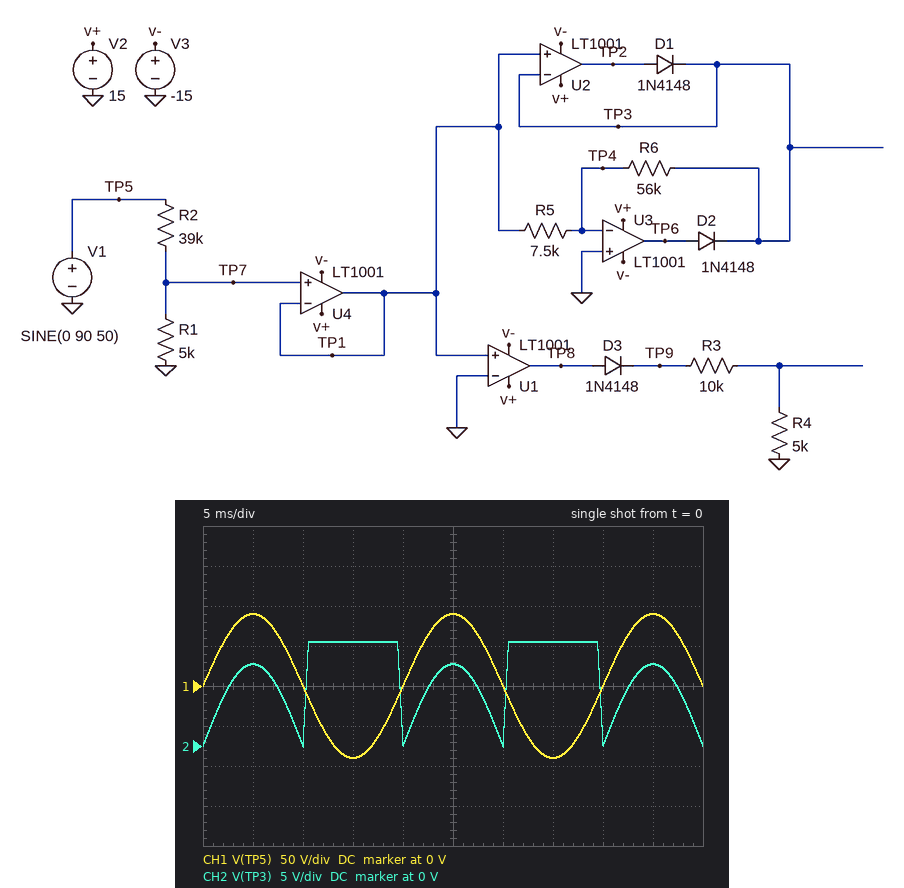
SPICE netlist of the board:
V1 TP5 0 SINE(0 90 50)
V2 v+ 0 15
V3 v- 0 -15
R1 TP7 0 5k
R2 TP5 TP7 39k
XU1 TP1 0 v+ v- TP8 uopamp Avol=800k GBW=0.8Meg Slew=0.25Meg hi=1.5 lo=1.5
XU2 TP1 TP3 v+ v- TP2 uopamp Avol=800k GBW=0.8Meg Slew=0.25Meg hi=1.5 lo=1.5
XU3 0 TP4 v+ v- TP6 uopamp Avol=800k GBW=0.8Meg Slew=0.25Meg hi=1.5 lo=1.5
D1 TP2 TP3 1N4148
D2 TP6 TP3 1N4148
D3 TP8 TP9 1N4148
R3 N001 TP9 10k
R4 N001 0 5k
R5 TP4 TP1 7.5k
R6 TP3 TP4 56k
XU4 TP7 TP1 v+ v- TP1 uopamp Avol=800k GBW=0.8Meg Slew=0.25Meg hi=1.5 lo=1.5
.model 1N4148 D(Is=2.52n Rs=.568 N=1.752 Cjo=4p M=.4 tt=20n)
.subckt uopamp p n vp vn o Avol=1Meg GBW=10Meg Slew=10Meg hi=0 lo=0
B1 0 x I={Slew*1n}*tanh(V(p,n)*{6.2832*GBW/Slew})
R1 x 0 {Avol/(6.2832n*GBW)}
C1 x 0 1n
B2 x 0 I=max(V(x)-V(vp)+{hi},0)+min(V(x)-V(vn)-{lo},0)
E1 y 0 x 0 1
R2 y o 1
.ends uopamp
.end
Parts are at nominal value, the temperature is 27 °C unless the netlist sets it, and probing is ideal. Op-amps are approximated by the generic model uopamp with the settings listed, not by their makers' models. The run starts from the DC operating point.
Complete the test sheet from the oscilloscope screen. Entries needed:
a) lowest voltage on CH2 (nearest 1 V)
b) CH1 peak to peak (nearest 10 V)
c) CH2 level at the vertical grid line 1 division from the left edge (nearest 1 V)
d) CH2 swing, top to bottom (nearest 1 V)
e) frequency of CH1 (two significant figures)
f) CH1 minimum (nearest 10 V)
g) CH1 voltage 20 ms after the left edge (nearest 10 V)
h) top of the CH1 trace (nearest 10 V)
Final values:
0 V
180 V
10 V
13 V
50 Hz
-90 V
0 V
90 V
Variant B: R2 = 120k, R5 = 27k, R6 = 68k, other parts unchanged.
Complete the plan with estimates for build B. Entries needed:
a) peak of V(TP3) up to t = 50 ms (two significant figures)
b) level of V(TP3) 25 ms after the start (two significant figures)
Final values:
9.1 V
3.6 V
